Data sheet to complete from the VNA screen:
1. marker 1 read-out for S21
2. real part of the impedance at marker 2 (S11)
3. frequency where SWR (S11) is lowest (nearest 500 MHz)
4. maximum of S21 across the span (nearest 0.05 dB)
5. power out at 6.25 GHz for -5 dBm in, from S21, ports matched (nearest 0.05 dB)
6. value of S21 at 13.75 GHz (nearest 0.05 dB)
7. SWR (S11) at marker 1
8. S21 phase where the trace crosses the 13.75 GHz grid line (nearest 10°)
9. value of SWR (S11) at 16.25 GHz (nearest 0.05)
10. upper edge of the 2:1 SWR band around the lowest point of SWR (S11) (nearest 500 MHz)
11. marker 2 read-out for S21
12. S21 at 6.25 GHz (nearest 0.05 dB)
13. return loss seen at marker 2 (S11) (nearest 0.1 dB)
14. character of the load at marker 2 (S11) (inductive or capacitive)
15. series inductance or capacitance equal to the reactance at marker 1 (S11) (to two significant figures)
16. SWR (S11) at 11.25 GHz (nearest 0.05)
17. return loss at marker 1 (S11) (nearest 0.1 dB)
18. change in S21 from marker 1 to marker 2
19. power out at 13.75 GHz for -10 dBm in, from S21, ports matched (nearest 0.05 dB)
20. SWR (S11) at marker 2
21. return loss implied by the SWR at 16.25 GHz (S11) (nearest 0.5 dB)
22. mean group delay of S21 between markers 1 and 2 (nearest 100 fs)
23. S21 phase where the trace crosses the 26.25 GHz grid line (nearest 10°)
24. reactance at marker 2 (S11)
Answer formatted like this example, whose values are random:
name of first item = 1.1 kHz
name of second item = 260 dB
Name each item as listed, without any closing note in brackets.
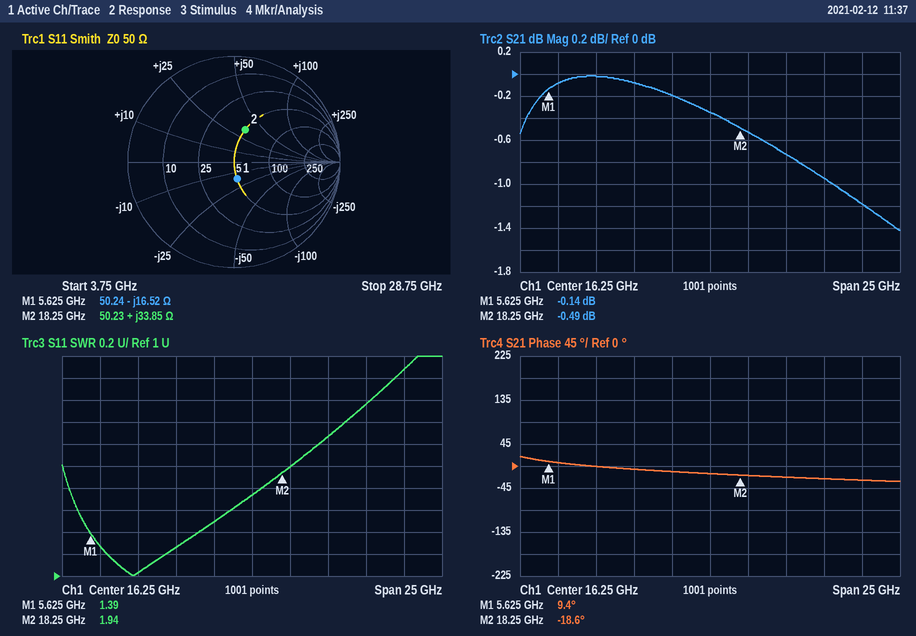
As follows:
marker 1 read-out for S21 = -0.14 dB
real part of the impedance at marker 2 = 50.23 Ω
frequency where SWR (S11) is lowest = 8.5 GHz
maximum of S21 across the span = 0.00 dB
power out at 6.25 GHz for -5 dBm in, from S21, ports matched = -5.10 dBm
value of S21 at 13.75 GHz = -0.20 dB
SWR (S11) at marker 1 = 1.39
S21 phase where the trace crosses the 13.75 GHz grid line = -10°
value of SWR (S11) at 16.25 GHz = 1.75
upper edge of the 2:1 SWR band around the lowest point of SWR (S11) = 19.0 GHz
marker 2 read-out for S21 = -0.49 dB
S21 at 6.25 GHz = -0.10 dB
return loss seen at marker 2 (S11) = 9.9 dB
character of the load at marker 2 (S11) = inductive
series inductance or capacitance equal to the reactance at marker 1 (S11) = 1.7 pF
SWR (S11) at 11.25 GHz = 1.25
return loss at marker 1 (S11) = 15.8 dB
change in S21 from marker 1 to marker 2 = -0.35 dB
power out at 13.75 GHz for -10 dBm in, from S21, ports matched = -10.20 dBm
SWR (S11) at marker 2 = 1.94
return loss implied by the SWR at 16.25 GHz (S11) = 11.5 dB
mean group delay of S21 between markers 1 and 2 = 6.2 ps
S21 phase where the trace crosses the 26.25 GHz grid line = -30°
reactance at marker 2 = +33.85 Ω
